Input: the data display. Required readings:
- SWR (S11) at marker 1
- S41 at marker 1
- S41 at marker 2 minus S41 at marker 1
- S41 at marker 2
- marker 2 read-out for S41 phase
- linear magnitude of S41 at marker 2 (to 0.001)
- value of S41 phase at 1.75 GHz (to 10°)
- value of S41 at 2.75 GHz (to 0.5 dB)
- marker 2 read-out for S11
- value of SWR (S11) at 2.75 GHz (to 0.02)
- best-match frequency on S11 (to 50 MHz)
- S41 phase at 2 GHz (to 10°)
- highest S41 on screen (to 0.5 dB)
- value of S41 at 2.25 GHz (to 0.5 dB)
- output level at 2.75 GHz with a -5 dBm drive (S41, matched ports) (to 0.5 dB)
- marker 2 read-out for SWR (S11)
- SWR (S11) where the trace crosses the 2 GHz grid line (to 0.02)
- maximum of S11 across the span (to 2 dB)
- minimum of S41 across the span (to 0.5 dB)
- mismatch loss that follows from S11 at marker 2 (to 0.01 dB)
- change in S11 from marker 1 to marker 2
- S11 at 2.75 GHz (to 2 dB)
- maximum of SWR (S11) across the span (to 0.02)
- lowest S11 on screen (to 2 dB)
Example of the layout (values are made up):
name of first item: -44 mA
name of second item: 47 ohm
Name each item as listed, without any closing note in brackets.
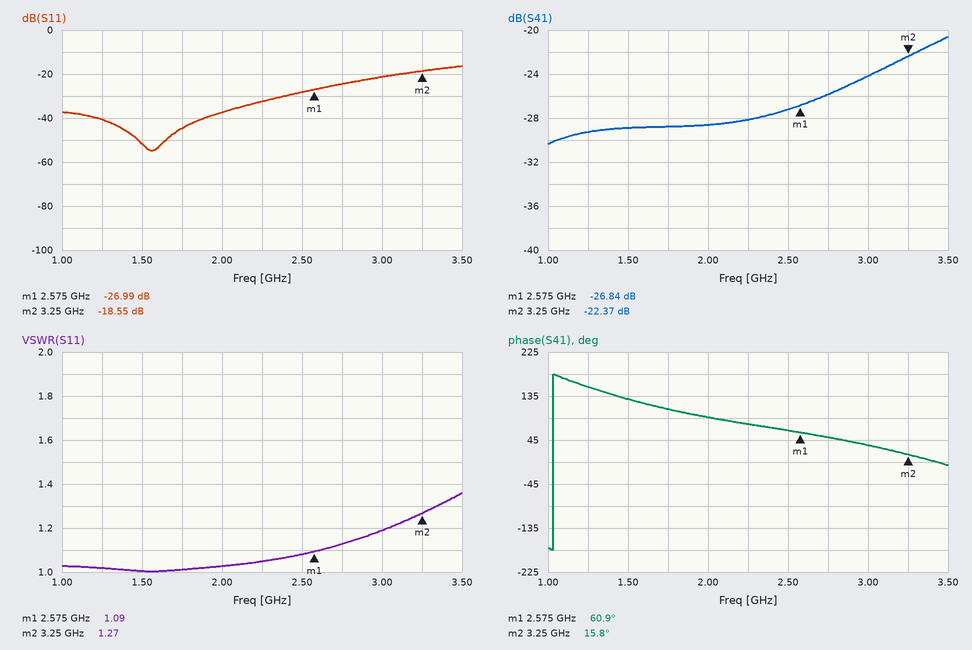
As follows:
SWR (S11) at marker 1: 1.09
S41 at marker 1: -26.84 dB
S41 at marker 2 minus S41 at marker 1: 4.47 dB
S41 at marker 2: -22.37 dB
marker 2 read-out for S41 phase: 15.8°
linear magnitude of S41 at marker 2: 0.076
value of S41 phase at 1.75 GHz: 110°
value of S41 at 2.75 GHz: -26.0 dB
marker 2 read-out for S11: -18.55 dB
value of SWR (S11) at 2.75 GHz: 1.12
best-match frequency on S11: 1.55 GHz
S41 phase at 2 GHz: 90°
highest S41 on screen: -20.5 dB
value of S41 at 2.25 GHz: -28.0 dB
output level at 2.75 GHz with a -5 dBm drive (S41, matched ports): -31.0 dBm
marker 2 read-out for SWR: 1.27
SWR (S11) where the trace crosses the 2 GHz grid line: 1.02
maximum of S11 across the span: -16 dB
minimum of S41 across the span: -30.5 dB
mismatch loss that follows from S11 at marker 2: 0.06 dB
change in S11 from marker 1 to marker 2: 8.44 dB
S11 at 2.75 GHz: -24 dB
maximum of SWR (S11) across the span: 1.36
lowest S11 on screen: -54 dB
